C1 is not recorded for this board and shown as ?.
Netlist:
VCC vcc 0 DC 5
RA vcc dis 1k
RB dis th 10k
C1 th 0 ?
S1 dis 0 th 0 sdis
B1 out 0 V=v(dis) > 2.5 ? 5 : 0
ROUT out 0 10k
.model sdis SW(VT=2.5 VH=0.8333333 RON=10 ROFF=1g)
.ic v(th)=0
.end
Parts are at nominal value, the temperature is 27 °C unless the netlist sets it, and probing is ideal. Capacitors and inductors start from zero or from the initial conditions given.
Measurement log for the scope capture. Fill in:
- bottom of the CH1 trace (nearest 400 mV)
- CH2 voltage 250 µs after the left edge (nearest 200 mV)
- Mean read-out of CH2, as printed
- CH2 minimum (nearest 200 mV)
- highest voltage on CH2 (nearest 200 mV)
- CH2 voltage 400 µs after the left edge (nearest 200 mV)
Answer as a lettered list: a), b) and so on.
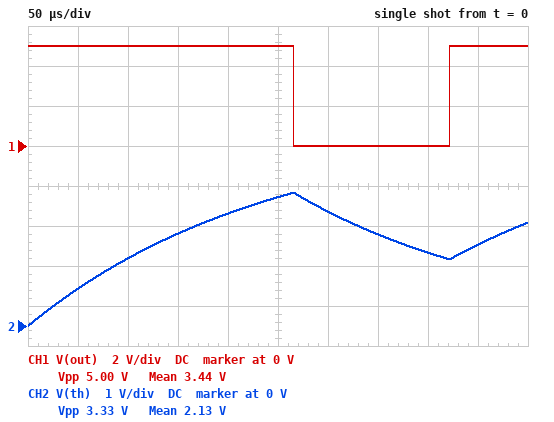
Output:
a) 0 V
b) 3.2 V
c) 2.13 V
d) 0 V
e) 3.4 V
f) 1.8 V
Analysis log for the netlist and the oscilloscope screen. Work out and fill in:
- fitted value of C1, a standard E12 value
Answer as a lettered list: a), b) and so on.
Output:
a) 22 nF
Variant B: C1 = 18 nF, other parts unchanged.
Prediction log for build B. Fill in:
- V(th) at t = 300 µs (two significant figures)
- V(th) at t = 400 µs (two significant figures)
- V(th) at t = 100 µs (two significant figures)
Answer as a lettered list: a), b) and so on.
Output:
a) 2.1 V
b) 2.5 V
c) 2.0 V
